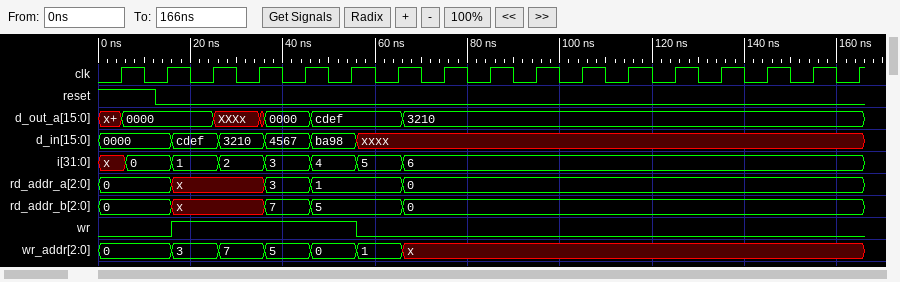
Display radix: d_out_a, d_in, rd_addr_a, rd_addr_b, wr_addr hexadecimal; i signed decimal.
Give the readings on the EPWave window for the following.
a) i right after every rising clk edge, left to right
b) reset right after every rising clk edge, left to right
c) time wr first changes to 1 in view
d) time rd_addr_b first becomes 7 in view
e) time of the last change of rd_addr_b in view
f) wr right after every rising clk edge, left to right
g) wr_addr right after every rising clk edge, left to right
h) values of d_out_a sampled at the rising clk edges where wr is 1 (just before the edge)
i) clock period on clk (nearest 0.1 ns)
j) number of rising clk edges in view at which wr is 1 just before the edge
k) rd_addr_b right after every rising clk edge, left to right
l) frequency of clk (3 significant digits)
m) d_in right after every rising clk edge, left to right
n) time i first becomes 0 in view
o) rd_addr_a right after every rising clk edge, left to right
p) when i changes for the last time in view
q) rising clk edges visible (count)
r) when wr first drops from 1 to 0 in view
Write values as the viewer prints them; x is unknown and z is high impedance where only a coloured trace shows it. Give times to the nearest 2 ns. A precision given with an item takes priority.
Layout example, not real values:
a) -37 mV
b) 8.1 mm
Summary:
a) x, 0, 1, 2, 3, 4, 5, 6, 6, 6, 6, 6, 6, 6, 6, 6, 6
b) 1 0 0 0 0 0 0 0 0 0 0 0 0 0 0 0 0
c) 16 ns
d) 36 ns
e) 66 ns
f) 0 0 1 1 1 1 0 0 0 0 0 0 0 0 0 0 0
g) 0, 0, 3, 7, 5, 0, 1, x, x, x, x, x, x, x, x, x, x
h) 0000, XXXx, 0000, cdef
i) 10 ns
j) 4
k) 0, 0, x, x, 7, 5, 5, 0, 0, 0, 0, 0, 0, 0, 0, 0, 0
l) 100 MHz
m) 0000, 0000, cdef, 3210, 4567, ba98, xxxx, xxxx, xxxx, xxxx, xxxx, xxxx, xxxx, xxxx, xxxx, xxxx, xxxx
n) 6 ns
o) 0, 0, x, x, 3, 1, 1, 0, 0, 0, 0, 0, 0, 0, 0, 0, 0
p) 66 ns
q) 17
r) 56 ns
